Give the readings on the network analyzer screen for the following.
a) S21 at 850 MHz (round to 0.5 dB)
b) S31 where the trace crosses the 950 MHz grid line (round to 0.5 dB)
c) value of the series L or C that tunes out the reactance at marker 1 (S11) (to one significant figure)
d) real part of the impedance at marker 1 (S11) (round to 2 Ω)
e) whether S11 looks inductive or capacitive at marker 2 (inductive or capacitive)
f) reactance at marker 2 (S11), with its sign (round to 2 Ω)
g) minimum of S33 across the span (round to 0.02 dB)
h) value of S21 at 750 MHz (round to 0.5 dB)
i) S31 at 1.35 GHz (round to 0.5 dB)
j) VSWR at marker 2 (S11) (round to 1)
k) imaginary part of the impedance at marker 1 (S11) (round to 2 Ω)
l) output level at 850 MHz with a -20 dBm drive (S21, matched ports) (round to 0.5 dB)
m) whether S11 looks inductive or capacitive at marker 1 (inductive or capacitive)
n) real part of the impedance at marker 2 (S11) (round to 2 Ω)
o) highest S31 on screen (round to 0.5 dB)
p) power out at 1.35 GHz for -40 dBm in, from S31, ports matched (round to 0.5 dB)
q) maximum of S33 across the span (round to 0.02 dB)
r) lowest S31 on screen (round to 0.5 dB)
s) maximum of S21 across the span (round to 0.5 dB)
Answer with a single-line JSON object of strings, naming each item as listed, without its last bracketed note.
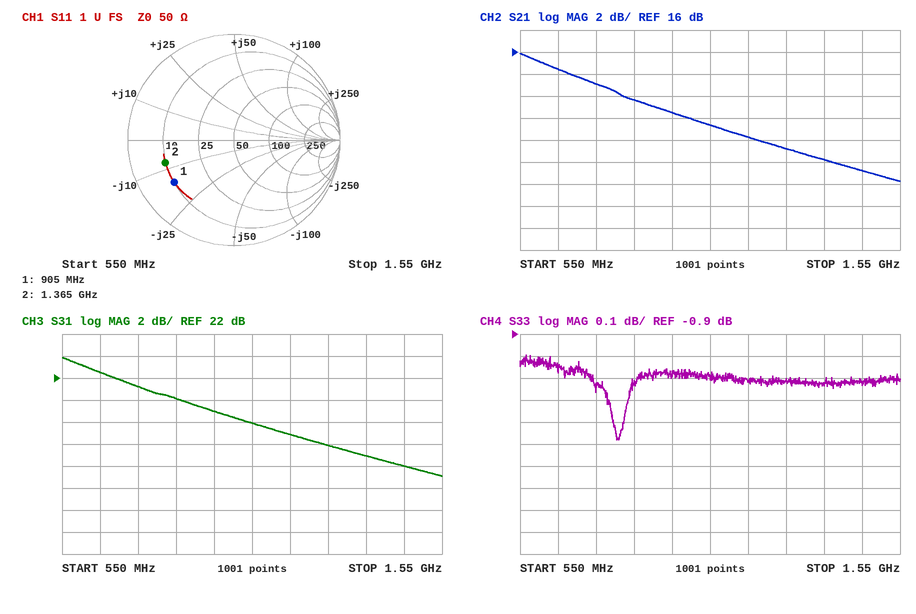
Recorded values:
{"S21 at 850 MHz": "11.5 dB", "S31 where the trace crosses the 950 MHz grid line": "19.0 dB", "value of the series L or C that tunes out the reactance at marker 1 (S11)": "3 nH", "real part of the impedance at marker 1 (S11)": "10 Ω", "whether S11 looks inductive or capacitive at marker 2": "capacitive", "reactance at marker 2 (S11), with its sign": "-8 Ω", "minimum of S33 across the span": "-1.38 dB", "value of S21 at 750 MHz": "13.0 dB", "S31 at 1.35 GHz": "15.0 dB", "VSWR at marker 2 (S11)": "5", "imaginary part of the impedance at marker 1 (S11)": "-16 Ω", "output level at 850 MHz with a -20 dBm drive (S21, matched ports)": "-8.5 dBm", "whether S11 looks inductive or capacitive at marker 1": "capacitive", "real part of the impedance at marker 2 (S11)": "10 Ω", "highest S31 on screen": "24.0 dB", "power out at 1.35 GHz for -40 dBm in, from S31, ports matched": "-25.0 dBm", "maximum of S33 across the span": "-1.00 dB", "lowest S31 on screen": "13.0 dB", "maximum of S21 across the span": "16.0 dB"}
